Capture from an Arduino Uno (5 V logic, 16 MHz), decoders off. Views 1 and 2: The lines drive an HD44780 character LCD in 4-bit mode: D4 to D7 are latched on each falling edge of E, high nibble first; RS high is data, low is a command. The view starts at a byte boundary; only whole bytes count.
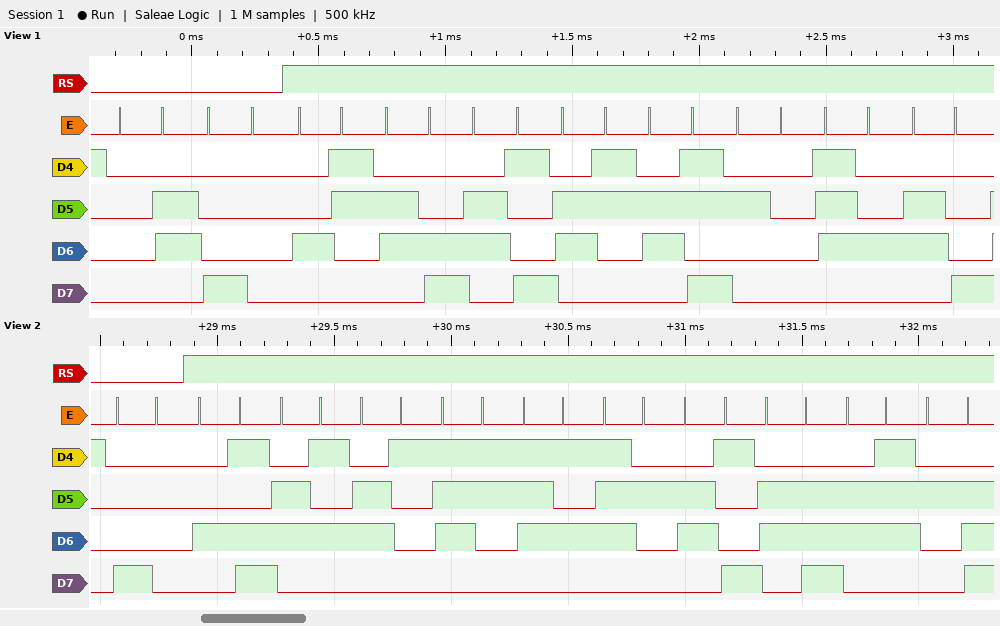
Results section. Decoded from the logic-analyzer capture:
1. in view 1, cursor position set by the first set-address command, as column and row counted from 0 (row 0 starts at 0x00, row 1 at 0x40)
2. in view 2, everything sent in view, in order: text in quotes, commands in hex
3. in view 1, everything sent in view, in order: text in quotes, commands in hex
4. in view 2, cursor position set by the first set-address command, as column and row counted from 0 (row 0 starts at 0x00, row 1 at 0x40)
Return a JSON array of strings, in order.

["column 0, row 0", "0x80 \"Measuring.\"", "0x06 0x80 \"Click th\"", "column 0, row 0"]
